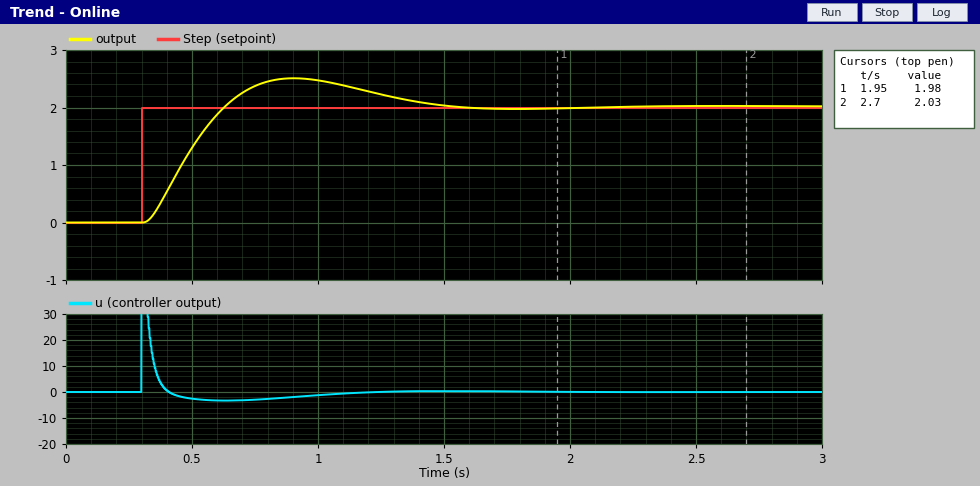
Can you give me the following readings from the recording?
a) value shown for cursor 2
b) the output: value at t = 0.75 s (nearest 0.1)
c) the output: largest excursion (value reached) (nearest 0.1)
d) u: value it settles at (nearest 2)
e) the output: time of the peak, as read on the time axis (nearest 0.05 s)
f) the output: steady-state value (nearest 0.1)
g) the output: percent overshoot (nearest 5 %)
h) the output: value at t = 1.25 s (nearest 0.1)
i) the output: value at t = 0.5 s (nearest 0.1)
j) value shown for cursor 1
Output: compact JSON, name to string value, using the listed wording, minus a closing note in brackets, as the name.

{"value shown for cursor 2": "2.03", "the output: value at t = 0.75 s": "2.4", "the output: largest excursion (value reached)": "2.5", "u: value it settles at": "0", "the output: time of the peak, as read on the time axis": "0.90 s", "the output: steady-state value": "2.0", "the output: percent overshoot": "25 %", "the output: value at t = 1.25 s": "2.2", "the output: value at t = 0.5 s": "1.3", "value shown for cursor 1": "1.98"}
